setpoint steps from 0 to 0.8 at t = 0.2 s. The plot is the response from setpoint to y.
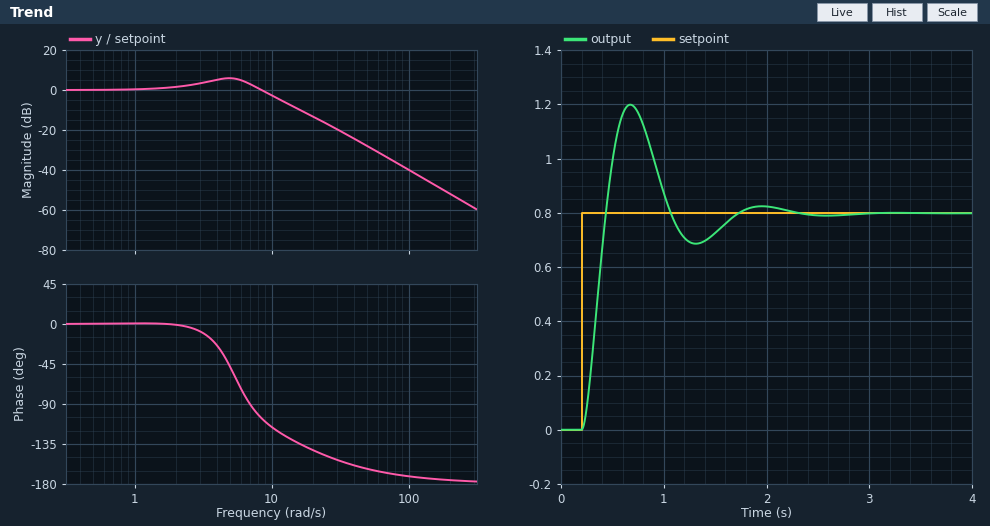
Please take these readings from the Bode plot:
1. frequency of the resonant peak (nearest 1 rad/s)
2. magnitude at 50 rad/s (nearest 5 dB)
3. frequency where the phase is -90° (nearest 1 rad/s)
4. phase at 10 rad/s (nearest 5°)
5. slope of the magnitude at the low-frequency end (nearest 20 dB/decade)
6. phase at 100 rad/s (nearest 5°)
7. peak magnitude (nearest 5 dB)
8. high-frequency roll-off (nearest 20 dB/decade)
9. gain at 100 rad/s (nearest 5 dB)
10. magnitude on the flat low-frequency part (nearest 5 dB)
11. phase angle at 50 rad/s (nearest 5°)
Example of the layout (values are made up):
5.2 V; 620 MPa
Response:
5 rad/s; -30 dB; 7 rad/s; -115°; 0 dB/decade; -170°; 5 dB; -40 dB/decade; -40 dB; 0 dB; -165°
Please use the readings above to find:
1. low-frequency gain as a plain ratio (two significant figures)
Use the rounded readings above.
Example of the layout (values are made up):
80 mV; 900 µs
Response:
1.0
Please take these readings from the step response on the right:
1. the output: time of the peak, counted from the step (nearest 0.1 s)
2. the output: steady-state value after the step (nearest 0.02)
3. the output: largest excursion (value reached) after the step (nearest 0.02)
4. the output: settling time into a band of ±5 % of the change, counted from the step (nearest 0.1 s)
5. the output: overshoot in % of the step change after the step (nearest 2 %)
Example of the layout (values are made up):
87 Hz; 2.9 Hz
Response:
0.5 s; 0.80; 1.20; 1.4 s; 50 %
